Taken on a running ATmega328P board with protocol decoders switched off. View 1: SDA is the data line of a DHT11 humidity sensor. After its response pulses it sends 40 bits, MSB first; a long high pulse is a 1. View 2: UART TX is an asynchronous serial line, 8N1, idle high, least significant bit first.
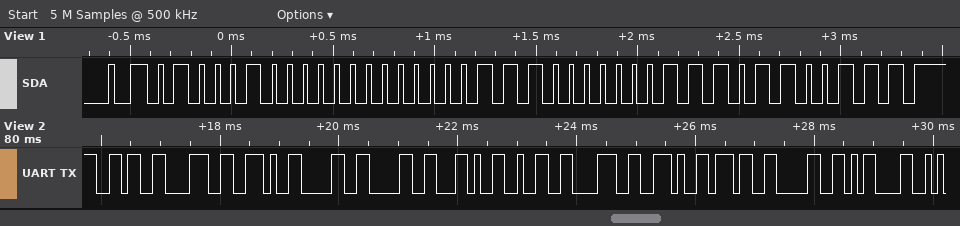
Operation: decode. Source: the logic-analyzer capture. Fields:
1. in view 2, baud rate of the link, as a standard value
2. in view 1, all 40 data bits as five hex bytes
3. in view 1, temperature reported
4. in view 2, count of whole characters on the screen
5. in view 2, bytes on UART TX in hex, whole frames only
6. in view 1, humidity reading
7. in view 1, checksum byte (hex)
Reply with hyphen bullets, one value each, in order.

- 9600 baud
- 44 00 1C 07 67
- 28.7 °C
- 12
- 36 38 2E 30 30 2C 32 38 2E 37 30 0D
- 68 %
- 0x67
